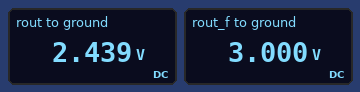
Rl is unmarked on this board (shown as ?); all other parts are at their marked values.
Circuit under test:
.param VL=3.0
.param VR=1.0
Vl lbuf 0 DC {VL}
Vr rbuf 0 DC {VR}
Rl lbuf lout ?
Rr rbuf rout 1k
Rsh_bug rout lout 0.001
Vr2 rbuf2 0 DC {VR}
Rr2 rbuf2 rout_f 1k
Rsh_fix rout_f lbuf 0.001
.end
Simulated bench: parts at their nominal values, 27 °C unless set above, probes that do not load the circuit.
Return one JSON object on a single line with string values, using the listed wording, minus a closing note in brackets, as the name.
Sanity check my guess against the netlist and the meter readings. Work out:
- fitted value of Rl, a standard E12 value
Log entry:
{"fitted value of Rl, a standard E12 value": "390 Ω"}
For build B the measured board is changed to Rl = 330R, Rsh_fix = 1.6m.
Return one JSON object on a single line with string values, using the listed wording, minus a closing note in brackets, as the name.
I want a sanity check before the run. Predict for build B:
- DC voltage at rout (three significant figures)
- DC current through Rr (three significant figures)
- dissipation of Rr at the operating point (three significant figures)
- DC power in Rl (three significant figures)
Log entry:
{"DC voltage at rout": "2.50 V", "DC current through Rr": "1.50 mA", "dissipation of Rr at the operating point": "2.26 mW", "DC power in Rl": "746 µW"}
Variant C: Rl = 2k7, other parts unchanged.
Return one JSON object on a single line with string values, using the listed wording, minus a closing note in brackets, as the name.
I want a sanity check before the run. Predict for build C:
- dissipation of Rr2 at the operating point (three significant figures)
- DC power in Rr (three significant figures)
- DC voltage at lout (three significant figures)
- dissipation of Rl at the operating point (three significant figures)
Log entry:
{"dissipation of Rr2 at the operating point": "4.00 mW", "DC power in Rr": "292 µW", "DC voltage at lout": "1.54 V", "dissipation of Rl at the operating point": "789 µW"}
